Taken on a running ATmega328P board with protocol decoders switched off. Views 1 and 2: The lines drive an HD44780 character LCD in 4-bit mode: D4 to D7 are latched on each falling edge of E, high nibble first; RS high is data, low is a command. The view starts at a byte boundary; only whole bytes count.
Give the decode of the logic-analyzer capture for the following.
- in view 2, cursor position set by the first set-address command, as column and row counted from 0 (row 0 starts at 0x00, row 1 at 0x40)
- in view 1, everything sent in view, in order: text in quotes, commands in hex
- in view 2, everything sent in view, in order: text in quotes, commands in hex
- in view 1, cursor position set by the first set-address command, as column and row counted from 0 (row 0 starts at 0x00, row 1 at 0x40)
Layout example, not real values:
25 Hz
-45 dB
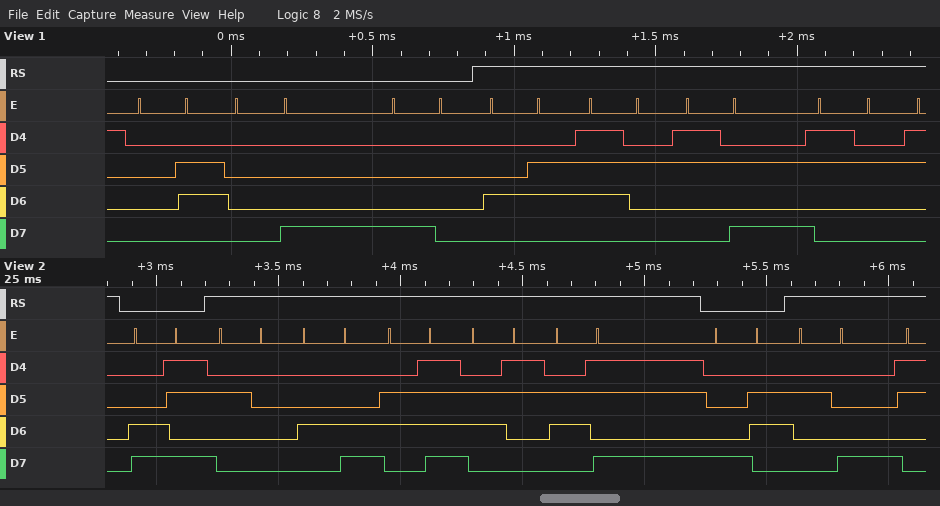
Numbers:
column 11, row 1
0x06 0x08 0x80 "Fr:2"
0xCB " Lock" 0x86 "("
column 0, row 0
